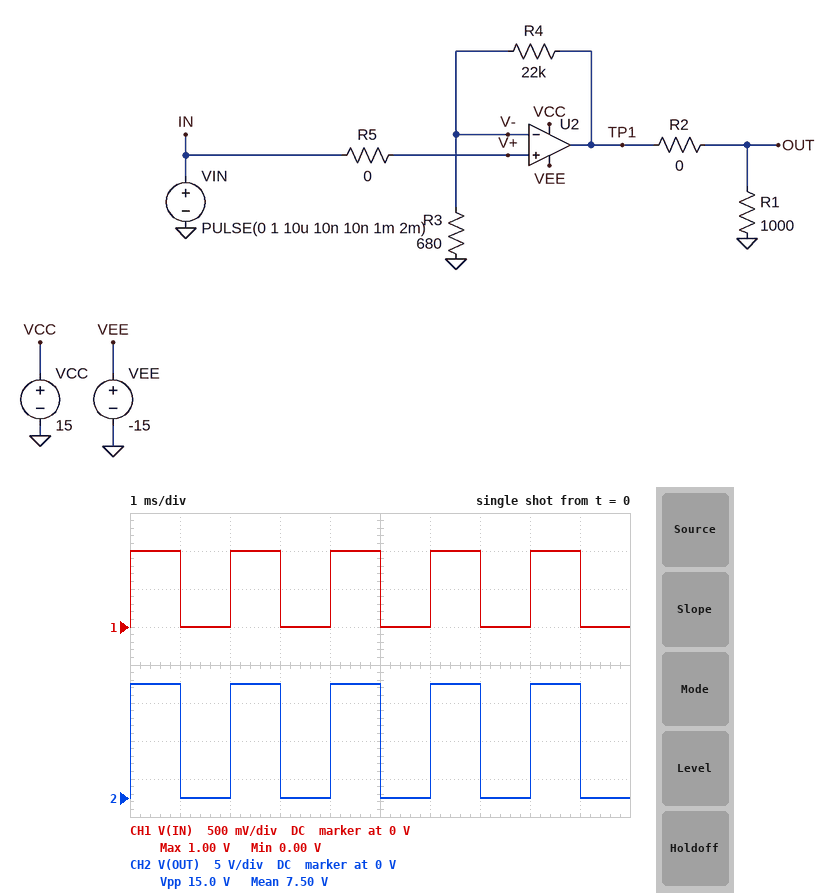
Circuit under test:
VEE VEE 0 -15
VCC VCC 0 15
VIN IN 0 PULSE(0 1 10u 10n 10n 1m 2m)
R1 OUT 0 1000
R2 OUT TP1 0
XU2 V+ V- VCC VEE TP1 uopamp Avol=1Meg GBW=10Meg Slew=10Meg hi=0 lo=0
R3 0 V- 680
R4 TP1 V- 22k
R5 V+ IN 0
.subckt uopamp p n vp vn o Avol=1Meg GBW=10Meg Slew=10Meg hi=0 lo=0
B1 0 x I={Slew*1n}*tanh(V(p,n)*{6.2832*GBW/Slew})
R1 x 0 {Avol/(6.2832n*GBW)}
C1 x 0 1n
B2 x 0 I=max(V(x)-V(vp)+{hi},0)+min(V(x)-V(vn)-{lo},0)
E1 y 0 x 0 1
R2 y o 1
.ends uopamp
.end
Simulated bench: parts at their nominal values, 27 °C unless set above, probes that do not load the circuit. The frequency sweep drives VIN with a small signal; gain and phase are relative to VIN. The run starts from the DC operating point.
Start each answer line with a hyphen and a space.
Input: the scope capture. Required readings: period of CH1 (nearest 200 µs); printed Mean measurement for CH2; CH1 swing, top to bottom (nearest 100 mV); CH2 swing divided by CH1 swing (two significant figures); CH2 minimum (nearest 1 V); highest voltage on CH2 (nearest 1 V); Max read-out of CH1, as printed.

- 2.0 ms
- 7.50 V
- 1.0 V
- 15
- 0 V
- 15 V
- 1.00 V
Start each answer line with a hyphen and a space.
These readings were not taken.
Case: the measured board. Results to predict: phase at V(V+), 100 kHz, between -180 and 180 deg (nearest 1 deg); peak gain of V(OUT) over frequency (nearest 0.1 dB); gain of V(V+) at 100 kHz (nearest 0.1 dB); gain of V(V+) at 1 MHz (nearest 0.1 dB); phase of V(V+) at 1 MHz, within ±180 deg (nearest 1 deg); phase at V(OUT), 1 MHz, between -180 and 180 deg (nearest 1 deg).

- 0 deg
- 30.5 dB
- 0 dB
- 0 dB
- 0 deg
- -73 deg
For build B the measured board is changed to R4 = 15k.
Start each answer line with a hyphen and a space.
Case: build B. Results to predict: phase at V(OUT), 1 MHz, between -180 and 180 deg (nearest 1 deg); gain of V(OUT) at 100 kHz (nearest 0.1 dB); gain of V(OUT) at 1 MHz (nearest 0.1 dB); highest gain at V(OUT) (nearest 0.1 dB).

- -67 deg
- 27.0 dB
- 19.2 dB
- 27.3 dB
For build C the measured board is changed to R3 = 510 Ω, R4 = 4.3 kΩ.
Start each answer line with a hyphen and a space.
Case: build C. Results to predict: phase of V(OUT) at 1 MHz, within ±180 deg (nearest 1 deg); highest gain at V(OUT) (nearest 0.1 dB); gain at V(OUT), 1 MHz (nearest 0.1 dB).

- -43 deg
- 19.5 dB
- 16.7 dB
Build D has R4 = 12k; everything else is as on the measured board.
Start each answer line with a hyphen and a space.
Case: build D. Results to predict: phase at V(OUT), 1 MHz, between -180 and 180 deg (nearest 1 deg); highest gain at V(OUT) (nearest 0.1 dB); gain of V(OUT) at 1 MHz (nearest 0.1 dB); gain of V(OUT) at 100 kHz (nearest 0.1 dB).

- -62 deg
- 25.4 dB
- 18.9 dB
- 25.3 dB
